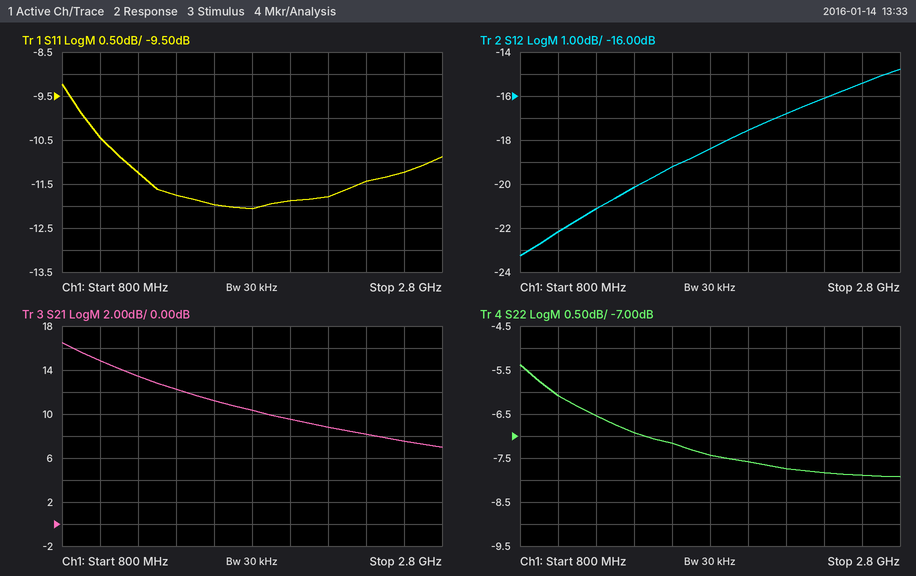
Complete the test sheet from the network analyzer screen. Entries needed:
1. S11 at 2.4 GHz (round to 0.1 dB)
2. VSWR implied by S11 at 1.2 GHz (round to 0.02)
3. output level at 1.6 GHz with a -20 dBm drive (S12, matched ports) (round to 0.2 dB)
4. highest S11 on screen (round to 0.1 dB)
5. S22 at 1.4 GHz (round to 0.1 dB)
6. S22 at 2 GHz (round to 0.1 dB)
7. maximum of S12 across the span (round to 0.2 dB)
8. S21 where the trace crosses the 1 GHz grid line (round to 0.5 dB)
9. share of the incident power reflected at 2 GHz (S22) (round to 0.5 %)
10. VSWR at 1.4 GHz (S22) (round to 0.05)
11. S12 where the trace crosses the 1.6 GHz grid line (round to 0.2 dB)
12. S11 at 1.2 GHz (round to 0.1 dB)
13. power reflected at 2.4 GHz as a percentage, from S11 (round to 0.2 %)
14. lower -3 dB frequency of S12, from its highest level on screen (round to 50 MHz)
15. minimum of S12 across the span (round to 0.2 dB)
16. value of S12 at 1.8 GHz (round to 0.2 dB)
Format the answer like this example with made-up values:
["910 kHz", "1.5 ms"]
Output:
["-11.4 dB", "1.76", "-39.2 dBm", "-9.2 dB", "-6.9 dB", "-7.6 dB", "-14.8 dB", "15.0 dB", "17.5 %", "2.65", "-19.2 dB", "-11.2 dB", "7.2 %", "1.95 GHz", "-23.2 dB", "-18.4 dB"]
